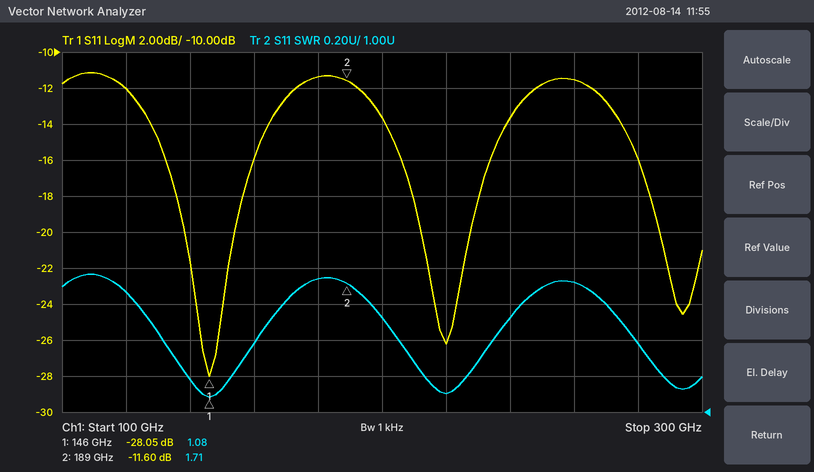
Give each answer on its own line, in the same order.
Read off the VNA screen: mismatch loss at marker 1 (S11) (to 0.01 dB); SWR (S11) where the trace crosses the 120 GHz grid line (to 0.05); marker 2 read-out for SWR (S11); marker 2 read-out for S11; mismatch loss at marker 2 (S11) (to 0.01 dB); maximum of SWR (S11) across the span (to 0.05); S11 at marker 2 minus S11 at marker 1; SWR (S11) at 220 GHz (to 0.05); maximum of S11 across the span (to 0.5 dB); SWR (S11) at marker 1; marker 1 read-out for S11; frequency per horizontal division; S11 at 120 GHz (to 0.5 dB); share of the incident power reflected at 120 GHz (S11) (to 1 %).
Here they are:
0.01 dB
1.65
1.71
-11.60 dB
0.31 dB
1.75
16.45 dB
1.10
-11.0 dB
1.08
-28.05 dB
20 GHz
-12.0 dB
6 %
